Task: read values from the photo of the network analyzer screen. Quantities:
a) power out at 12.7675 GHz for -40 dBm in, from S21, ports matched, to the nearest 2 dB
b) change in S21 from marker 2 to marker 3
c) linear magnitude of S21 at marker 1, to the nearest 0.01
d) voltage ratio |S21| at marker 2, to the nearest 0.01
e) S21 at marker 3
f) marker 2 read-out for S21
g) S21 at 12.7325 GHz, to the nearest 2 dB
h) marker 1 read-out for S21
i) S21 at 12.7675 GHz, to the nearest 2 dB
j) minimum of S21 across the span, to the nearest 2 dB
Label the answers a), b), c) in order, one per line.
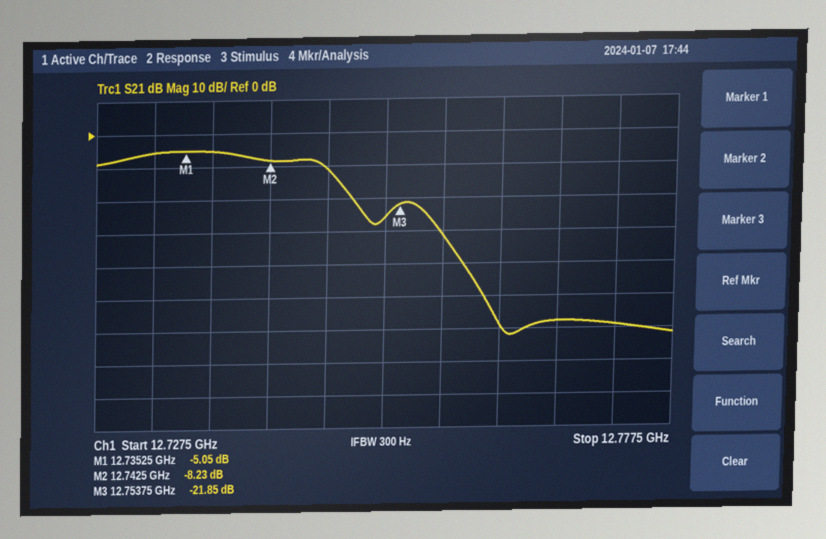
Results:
a) -98 dBm
b) -13.62 dB
c) 0.56
d) 0.39
e) -21.85 dB
f) -8.23 dB
g) -6 dB
h) -5.05 dB
i) -58 dB
j) -62 dB
